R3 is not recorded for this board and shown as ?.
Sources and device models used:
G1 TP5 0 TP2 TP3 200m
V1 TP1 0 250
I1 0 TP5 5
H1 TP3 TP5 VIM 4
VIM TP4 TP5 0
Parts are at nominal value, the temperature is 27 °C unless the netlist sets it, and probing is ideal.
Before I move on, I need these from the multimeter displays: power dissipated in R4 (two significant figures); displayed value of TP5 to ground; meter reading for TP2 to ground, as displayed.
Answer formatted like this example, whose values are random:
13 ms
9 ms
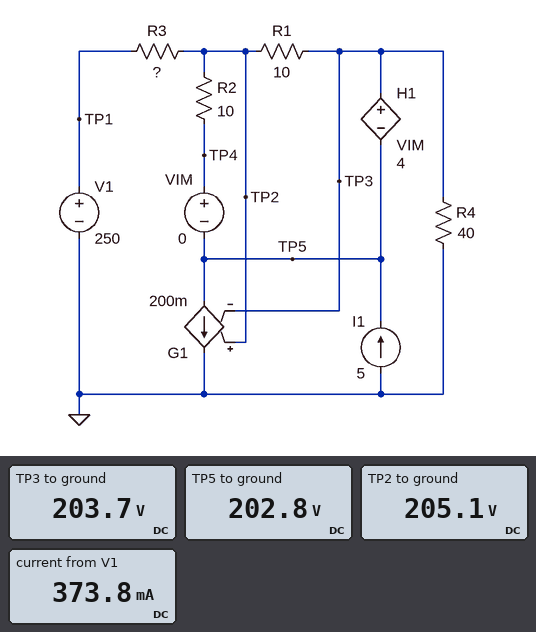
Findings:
1.0 kW
202.8 V
205.1 V
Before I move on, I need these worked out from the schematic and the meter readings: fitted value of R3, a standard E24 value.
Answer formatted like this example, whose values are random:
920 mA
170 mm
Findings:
120 Ω
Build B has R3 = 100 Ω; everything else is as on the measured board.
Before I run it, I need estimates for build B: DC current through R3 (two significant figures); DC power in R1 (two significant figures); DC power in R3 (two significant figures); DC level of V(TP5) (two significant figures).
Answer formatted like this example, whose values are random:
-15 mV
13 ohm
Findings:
440 mA
270 mW
19 W
200 V
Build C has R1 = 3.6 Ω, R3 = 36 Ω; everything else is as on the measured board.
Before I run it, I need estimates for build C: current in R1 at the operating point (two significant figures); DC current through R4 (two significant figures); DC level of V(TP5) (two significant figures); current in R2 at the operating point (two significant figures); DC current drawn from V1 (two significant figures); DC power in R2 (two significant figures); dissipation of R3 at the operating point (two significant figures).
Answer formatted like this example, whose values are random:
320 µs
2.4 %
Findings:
520 mA
5.5 A
220 V
310 mA
830 mA
970 mW
25 W
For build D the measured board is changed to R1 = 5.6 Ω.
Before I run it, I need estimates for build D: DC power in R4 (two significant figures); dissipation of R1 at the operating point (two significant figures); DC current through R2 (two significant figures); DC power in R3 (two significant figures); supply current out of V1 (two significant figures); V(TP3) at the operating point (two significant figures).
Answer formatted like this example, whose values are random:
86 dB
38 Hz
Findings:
1.1 kW
190 mW
170 mA
15 W
360 mA
210 V
